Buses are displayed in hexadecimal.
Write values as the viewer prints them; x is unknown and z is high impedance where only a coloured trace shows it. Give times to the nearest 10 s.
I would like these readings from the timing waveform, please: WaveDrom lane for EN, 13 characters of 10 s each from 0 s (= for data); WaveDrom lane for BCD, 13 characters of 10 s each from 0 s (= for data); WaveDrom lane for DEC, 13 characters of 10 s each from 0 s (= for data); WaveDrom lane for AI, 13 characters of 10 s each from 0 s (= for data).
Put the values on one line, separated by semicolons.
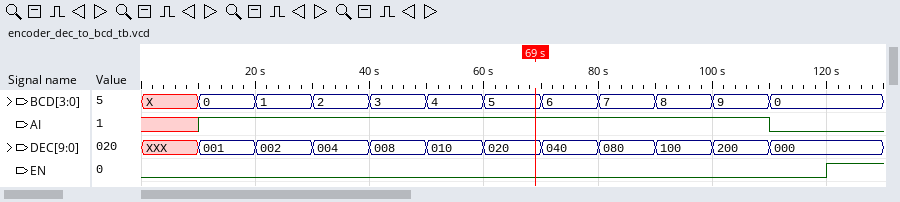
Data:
{name: 'EN', wave: '0...........1'}; {name: 'BCD', wave: 'x===========.', data: '0 1 2 3 4 5 6 7 8 9 0'}; {name: 'DEC', wave: 'x===========.', data: '001 002 004 008 010 020 040 080 100 200 000'}; {name: 'AI', wave: 'x1.........0.'}
